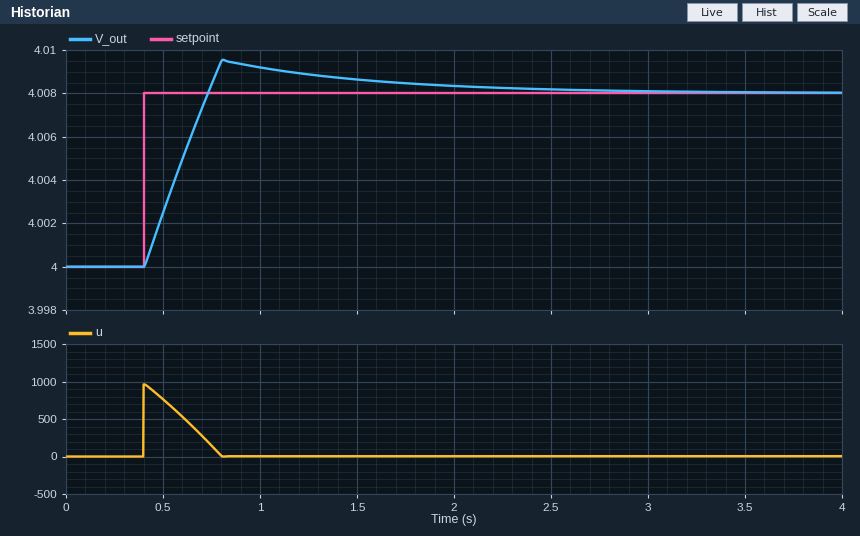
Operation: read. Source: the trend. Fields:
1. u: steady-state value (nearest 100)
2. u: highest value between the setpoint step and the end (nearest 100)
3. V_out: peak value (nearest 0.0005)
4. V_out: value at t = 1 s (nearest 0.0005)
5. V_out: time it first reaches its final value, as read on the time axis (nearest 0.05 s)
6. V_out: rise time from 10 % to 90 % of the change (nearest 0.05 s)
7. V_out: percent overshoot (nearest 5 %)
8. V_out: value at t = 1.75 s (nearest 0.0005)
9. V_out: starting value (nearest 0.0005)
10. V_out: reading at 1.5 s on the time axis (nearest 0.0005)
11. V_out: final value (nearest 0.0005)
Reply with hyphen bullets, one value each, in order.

- 0
- 1000
- 4.0095
- 4.0090
- 0.75 s
- 0.25 s
- 20 %
- 4.0085
- 4.0000
- 4.0085
- 4.0080
